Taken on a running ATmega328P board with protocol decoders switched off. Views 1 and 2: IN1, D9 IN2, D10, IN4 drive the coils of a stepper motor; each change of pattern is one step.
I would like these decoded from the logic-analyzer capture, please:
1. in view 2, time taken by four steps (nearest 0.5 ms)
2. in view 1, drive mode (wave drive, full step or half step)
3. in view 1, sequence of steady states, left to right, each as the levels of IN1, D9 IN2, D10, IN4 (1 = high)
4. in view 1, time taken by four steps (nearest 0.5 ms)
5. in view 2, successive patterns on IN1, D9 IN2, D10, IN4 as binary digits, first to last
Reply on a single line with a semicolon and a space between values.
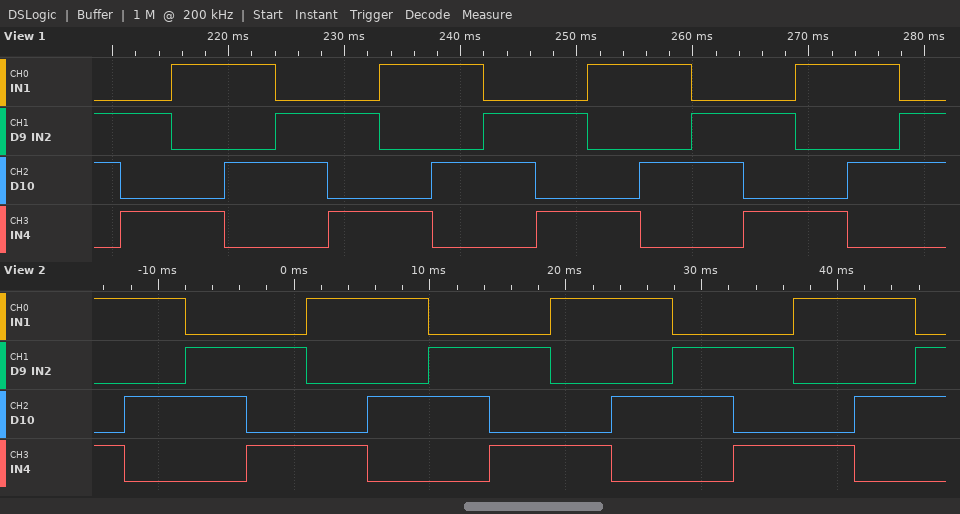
18.0 ms; full step; 0110 0101 1001 1010 0110 0101 1001 1010 0110 0101 1001 1010 0110 0101 1001 1010 0110; 18.0 ms; 1001 1010 0110 0101 1001 1010 0110 0101 1001 1010 0110 0101 1001 1010 0110
